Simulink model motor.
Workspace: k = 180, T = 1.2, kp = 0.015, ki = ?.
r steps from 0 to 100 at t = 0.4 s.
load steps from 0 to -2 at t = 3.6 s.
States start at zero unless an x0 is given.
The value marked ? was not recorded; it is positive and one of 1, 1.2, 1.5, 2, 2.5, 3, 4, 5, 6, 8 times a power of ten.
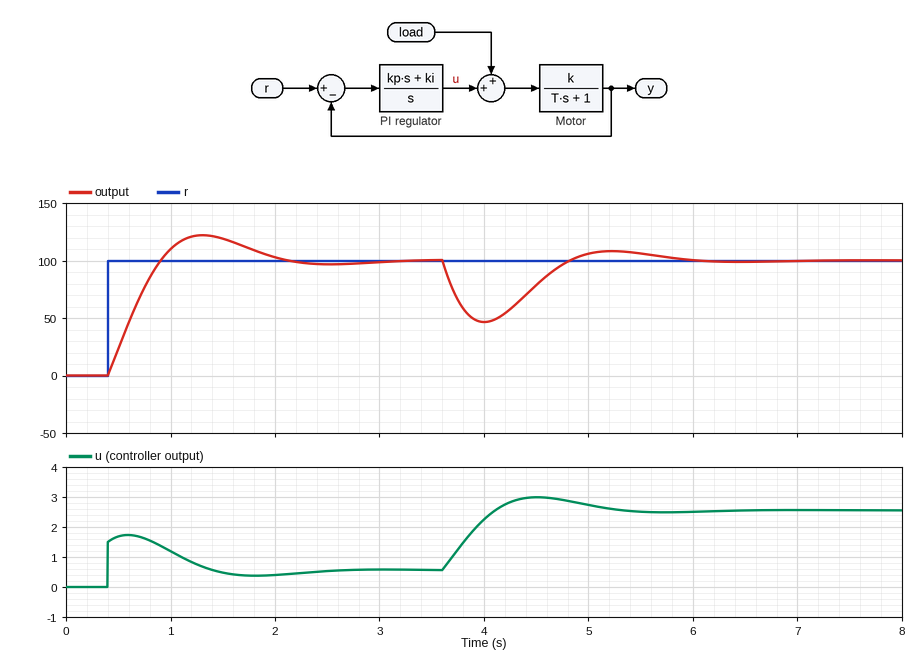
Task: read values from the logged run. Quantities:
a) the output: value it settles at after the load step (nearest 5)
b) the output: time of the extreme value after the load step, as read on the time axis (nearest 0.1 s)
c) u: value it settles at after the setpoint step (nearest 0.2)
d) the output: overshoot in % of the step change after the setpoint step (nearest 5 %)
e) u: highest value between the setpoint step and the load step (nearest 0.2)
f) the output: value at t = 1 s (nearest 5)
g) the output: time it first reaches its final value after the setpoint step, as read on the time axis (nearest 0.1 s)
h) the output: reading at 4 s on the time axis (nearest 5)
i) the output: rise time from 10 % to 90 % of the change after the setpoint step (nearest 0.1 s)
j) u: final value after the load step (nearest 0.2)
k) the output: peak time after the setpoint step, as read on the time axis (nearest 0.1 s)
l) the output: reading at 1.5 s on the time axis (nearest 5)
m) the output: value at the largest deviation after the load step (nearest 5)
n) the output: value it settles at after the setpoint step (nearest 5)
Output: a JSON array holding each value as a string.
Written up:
["100", "4.0 s", "0.6", "20 %", "1.8", "110", "0.9 s", "45", "0.4 s", "2.6", "1.3 s", "120", "45", "100"]
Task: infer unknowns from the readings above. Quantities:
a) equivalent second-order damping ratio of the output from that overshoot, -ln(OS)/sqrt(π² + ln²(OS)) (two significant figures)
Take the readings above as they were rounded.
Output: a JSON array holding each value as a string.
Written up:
["0.46"]
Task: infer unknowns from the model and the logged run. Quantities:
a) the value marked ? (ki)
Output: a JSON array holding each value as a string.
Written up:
["0.06"]
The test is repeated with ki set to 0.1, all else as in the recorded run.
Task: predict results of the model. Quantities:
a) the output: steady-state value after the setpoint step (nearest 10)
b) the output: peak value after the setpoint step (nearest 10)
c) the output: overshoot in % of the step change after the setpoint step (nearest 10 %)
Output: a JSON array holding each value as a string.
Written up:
["100", "130", "30 %"]
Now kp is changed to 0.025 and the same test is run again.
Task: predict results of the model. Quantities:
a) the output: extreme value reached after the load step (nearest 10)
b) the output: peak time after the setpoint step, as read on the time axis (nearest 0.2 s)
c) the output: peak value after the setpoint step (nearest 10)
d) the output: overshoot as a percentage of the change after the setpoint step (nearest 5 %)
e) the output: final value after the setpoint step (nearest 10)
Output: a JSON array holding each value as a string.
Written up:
["60", "1.2 s", "110", "10 %", "100"]
